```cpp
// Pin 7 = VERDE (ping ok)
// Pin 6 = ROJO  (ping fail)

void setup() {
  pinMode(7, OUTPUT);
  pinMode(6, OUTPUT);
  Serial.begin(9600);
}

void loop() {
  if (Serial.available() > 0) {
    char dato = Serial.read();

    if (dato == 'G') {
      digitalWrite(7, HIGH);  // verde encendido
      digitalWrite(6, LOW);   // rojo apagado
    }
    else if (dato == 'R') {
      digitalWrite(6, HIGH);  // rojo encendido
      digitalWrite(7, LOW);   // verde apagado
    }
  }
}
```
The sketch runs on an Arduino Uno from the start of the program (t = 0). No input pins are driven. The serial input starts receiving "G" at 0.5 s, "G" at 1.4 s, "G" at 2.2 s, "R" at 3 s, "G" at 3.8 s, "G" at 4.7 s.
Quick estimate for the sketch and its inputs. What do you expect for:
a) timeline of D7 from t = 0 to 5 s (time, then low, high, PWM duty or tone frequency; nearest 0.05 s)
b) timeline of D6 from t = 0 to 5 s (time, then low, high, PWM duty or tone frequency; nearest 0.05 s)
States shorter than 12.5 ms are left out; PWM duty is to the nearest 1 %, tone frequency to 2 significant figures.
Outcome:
0 s low; 0.5 s high; 3 s low; 3.8 s high
0 s low; 3 s high; 3.8 s low
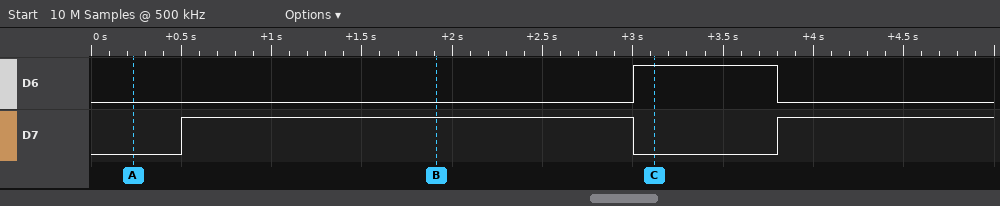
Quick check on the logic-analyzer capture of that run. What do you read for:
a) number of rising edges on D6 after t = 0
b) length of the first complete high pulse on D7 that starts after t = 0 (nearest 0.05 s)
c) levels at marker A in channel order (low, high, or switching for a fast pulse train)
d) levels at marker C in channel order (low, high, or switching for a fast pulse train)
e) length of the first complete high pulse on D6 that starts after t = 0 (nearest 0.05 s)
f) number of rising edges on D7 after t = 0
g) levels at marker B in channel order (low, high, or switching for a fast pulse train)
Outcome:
1
2.50 s
D6 low, D7 low
D6 high, D7 low
0.80 s
2
D6 low, D7 high
